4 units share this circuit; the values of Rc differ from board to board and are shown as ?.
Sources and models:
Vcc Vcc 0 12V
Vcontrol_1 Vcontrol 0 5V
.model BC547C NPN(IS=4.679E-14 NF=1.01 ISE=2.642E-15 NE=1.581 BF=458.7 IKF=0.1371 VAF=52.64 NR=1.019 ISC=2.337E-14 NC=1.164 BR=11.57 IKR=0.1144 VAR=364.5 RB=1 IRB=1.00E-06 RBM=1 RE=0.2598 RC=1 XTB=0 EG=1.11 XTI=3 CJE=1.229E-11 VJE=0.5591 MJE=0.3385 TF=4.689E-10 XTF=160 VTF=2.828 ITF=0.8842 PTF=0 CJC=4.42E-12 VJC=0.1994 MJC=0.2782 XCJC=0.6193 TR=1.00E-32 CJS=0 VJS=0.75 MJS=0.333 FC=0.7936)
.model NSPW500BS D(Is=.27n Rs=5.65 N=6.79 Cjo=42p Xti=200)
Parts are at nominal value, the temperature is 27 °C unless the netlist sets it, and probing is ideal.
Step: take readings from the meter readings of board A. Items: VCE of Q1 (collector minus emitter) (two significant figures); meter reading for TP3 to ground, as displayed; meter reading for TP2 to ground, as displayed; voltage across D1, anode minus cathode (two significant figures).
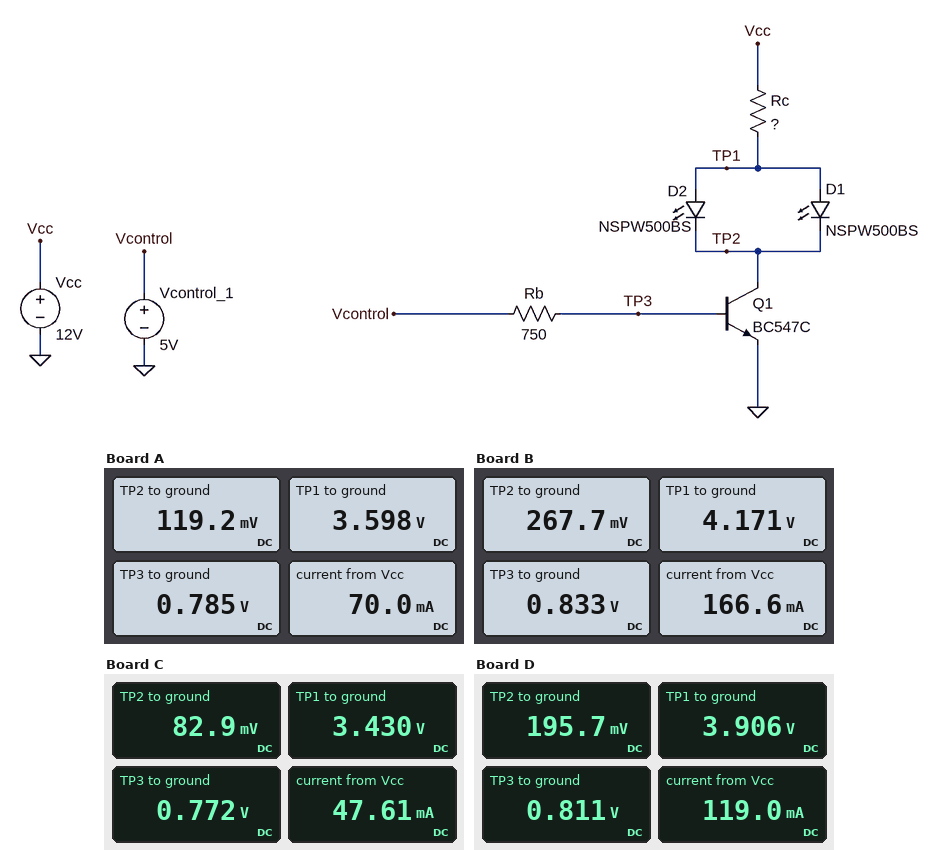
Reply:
120 mV
0.785 V
119.2 mV
3.5 V
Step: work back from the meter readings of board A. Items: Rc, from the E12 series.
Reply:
120 Ω
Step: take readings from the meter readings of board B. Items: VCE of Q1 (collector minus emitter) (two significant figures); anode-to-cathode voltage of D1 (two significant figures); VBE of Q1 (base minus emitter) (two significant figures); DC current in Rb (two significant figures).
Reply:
270 mV
3.9 V
830 mV
5.6 mA
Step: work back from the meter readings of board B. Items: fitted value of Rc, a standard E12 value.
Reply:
47 Ω
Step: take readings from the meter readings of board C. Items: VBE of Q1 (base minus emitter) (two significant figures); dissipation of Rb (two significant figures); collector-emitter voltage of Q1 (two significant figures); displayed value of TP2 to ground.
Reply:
770 mV
24 mW
83 mV
82.9 mV
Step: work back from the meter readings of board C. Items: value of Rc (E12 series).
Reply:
180 Ω
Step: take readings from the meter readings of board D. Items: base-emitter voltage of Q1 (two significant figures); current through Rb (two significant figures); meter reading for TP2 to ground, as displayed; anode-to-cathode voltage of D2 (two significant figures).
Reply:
810 mV
5.6 mA
195.7 mV
3.7 V
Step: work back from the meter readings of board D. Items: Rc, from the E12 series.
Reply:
68 Ω
